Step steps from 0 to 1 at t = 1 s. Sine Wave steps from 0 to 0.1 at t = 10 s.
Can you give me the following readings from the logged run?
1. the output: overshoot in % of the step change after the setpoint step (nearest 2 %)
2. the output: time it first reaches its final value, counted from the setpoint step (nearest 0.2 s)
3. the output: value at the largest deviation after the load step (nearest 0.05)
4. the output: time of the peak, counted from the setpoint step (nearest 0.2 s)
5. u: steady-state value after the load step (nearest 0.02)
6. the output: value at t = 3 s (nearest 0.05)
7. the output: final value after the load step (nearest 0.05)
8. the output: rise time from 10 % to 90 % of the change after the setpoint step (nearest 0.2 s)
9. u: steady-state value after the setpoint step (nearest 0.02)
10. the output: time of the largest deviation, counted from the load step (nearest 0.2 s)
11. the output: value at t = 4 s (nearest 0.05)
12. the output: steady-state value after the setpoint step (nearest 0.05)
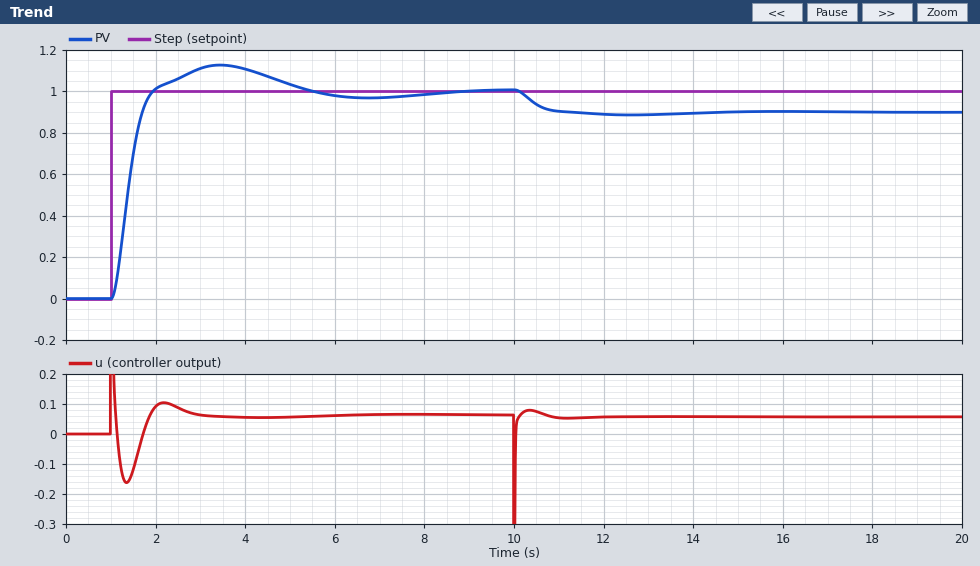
12 %
1.0 s
0.90
2.4 s
0.06
1.10
0.90
0.6 s
0.06
2.6 s
1.10
1.00
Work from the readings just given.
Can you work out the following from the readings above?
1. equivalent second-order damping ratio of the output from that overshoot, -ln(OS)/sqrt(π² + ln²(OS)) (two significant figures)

0.56
